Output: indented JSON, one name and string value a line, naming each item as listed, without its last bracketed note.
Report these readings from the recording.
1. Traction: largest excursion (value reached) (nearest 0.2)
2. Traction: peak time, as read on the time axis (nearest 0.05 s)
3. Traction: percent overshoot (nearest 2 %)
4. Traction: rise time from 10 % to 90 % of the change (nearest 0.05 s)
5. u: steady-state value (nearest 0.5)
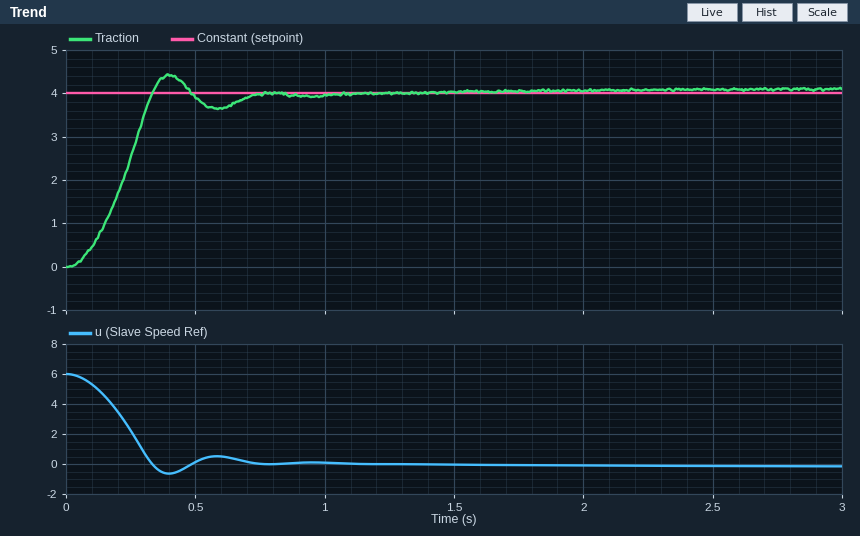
{
  "Traction: largest excursion (value reached)": "4.4",
  "Traction: peak time, as read on the time axis": "0.40 s",
  "Traction: percent overshoot": "8 %",
  "Traction: rise time from 10 % to 90 % of the change": "0.20 s",
  "u: steady-state value": "0.0"
}
